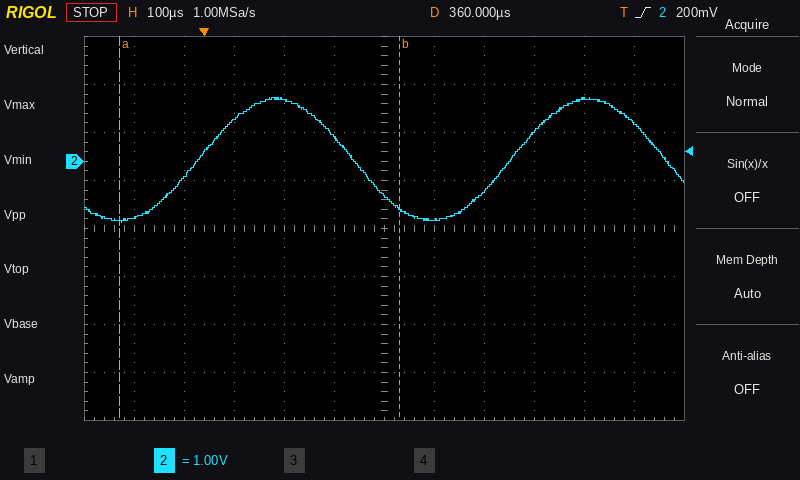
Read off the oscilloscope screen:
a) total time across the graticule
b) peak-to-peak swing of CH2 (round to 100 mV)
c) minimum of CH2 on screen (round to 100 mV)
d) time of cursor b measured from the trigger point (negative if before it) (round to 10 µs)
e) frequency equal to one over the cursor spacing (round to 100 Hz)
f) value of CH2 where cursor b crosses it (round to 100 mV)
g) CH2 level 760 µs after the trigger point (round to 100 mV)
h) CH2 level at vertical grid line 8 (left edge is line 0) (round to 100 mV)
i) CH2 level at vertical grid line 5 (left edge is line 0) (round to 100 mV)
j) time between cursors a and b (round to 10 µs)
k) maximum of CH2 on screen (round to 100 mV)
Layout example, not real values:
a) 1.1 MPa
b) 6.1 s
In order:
a) 1.2 ms
b) 2.6 V
c) -1.3 V
d) +390 µs
e) 1.8 kHz
f) -1.0 V
g) 1.3 V
h) -600 mV
i) 500 mV
j) 560 µs
k) 1.3 V
